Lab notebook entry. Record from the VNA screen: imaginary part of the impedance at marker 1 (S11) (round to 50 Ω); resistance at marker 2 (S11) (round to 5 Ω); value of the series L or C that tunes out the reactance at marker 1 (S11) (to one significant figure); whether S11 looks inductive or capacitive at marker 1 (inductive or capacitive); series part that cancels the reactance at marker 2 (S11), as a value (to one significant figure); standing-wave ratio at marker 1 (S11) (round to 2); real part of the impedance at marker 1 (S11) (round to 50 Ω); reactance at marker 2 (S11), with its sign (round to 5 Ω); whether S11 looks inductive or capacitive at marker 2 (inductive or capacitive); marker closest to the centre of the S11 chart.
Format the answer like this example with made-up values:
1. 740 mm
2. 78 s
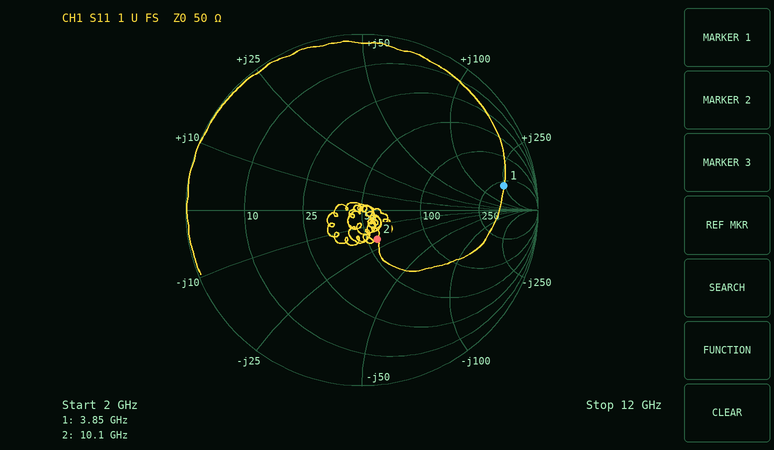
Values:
1. +250 Ω
2. 55 Ω
3. 200 fF
4. inductive
5. 300 pH
6. 10
7. 300 Ω
8. -20 Ω
9. capacitive
10. marker 2
